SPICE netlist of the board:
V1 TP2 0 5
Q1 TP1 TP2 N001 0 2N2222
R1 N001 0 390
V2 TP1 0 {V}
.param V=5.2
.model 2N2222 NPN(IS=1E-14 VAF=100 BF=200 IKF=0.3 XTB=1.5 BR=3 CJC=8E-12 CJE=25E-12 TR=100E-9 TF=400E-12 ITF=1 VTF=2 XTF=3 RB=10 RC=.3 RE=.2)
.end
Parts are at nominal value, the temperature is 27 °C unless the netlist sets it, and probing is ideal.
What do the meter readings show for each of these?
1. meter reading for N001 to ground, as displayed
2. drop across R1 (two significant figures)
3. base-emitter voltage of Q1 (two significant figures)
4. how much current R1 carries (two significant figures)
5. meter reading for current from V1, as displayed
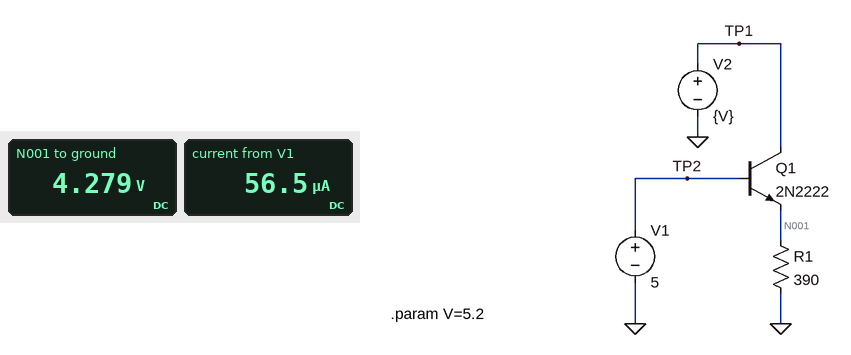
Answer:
4.279 V
4.3 V
720 mV
11 mA
56.5 µA
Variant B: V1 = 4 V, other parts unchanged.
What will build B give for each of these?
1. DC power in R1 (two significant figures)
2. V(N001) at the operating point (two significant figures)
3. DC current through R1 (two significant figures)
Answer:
28 mW
3.3 V
8.4 mA
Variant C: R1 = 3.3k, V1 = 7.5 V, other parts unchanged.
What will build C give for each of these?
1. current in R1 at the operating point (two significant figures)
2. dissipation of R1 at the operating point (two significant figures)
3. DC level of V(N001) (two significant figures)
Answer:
1.6 mA
8.3 mW
5.2 V
